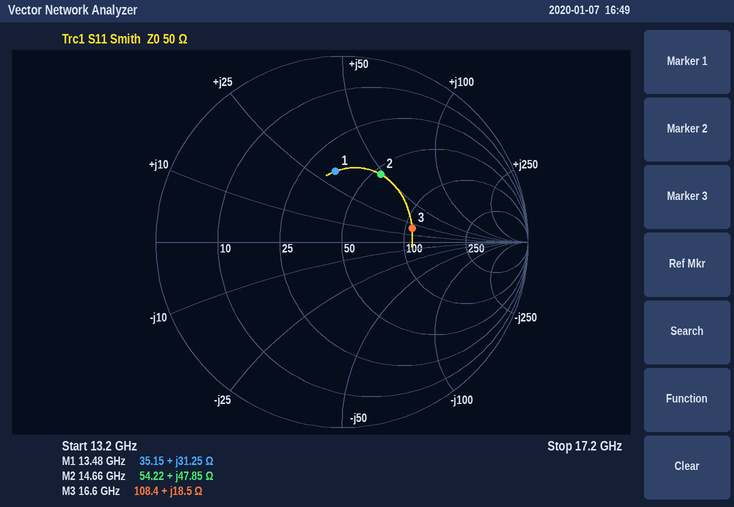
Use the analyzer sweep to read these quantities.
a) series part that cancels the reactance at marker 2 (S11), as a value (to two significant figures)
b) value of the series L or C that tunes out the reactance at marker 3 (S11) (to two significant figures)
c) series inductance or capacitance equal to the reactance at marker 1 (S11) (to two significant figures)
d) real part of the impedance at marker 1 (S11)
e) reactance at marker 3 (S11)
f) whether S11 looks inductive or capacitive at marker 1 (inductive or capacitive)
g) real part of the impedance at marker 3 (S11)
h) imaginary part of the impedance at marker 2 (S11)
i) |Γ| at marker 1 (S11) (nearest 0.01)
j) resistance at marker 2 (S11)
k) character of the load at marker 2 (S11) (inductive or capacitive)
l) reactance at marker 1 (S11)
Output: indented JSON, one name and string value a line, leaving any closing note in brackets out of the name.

{
  "series part that cancels the reactance at marker 2 (S11), as a value": "230 fF",
  "value of the series L or C that tunes out the reactance at marker 3 (S11)": "520 fF",
  "series inductance or capacitance equal to the reactance at marker 1 (S11)": "370 pH",
  "real part of the impedance at marker 1": "35.15 Ω",
  "reactance at marker 3": "+18.5 Ω",
  "whether S11 looks inductive or capacitive at marker 1": "inductive",
  "real part of the impedance at marker 3": "108.4 Ω",
  "imaginary part of the impedance at marker 2": "+47.85 Ω",
  "|Γ| at marker 1 (S11)": "0.38",
  "resistance at marker 2": "54.22 Ω",
  "character of the load at marker 2 (S11)": "inductive",
  "reactance at marker 1": "+31.25 Ω"
}
